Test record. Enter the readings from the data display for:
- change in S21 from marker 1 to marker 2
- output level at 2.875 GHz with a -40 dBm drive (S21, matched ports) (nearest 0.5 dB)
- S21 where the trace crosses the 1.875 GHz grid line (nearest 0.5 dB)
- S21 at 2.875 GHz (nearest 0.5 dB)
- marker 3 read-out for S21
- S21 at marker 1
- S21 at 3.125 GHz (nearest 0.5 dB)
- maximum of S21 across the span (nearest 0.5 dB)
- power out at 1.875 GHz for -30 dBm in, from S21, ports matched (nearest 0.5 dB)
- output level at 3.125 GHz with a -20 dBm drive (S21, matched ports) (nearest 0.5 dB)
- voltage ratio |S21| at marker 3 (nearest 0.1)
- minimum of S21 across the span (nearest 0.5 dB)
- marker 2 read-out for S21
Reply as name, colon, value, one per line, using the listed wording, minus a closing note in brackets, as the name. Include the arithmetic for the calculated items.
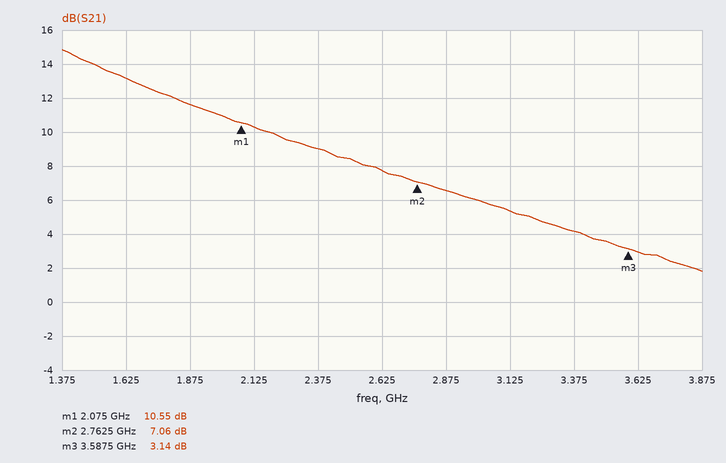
change in S21 from marker 1 to marker 2: 7.06 − (10.55) = -3.49 dB
output level at 2.875 GHz with a -40 dBm drive (S21, matched ports): -40 dBm + (6.5 dB) = -33.5 dBm
S21 where the trace crosses the 1.875 GHz grid line: 11.5 dB
S21 at 2.875 GHz: 6.5 dB
marker 3 read-out for S21: 3.14 dB
S21 at marker 1: 10.55 dB
S21 at 3.125 GHz: 5.5 dB
maximum of S21 across the span: 15.0 dB
power out at 1.875 GHz for -30 dBm in, from S21, ports matched: -30 dBm + (11.5 dB) = -18.5 dBm
output level at 3.125 GHz with a -20 dBm drive (S21, matched ports): -20 dBm + (5.5 dB) = -14.5 dBm
voltage ratio |S21| at marker 3: 10^(3.14/20) ≈ 1.4
minimum of S21 across the span: 2.0 dB
marker 2 read-out for S21: 7.06 dB
